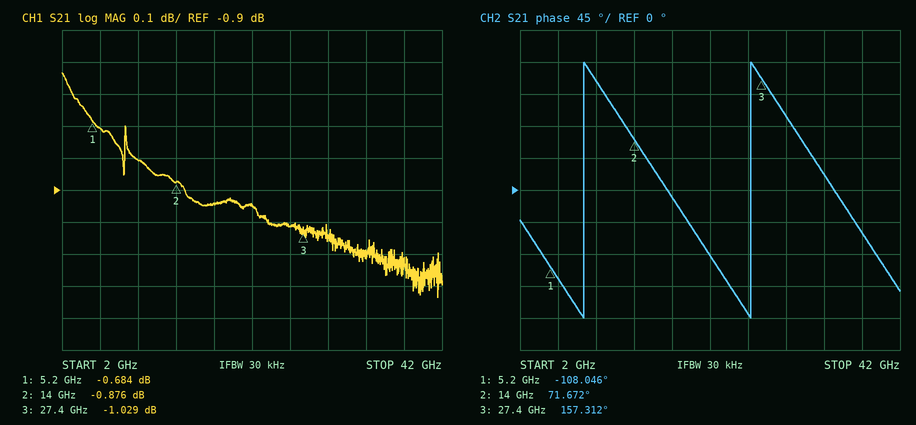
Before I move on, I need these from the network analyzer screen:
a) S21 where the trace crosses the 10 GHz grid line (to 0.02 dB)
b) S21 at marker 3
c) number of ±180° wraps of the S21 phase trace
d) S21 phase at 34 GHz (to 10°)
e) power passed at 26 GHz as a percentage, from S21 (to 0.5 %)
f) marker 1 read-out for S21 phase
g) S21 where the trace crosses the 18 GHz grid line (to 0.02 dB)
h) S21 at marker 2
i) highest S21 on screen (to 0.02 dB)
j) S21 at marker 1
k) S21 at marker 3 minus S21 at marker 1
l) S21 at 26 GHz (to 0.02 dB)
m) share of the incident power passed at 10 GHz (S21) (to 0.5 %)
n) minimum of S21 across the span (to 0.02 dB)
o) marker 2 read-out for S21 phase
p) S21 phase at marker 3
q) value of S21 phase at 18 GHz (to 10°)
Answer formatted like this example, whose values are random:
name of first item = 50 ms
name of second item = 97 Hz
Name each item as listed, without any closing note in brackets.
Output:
S21 where the trace crosses the 10 GHz grid line = -0.80 dB
S21 at marker 3 = -1.029 dB
number of ±180° wraps of the S21 phase trace = 2
S21 phase at 34 GHz = 20°
power passed at 26 GHz as a percentage, from S21 = 79.0 %
marker 1 read-out for S21 phase = -108.046°
S21 where the trace crosses the 18 GHz grid line = -0.94 dB
S21 at marker 2 = -0.876 dB
highest S21 on screen = -0.54 dB
S21 at marker 1 = -0.684 dB
S21 at marker 3 minus S21 at marker 1 = -0.345 dB
S21 at 26 GHz = -1.02 dB
share of the incident power passed at 10 GHz (S21) = 83.0 %
minimum of S21 across the span = -1.24 dB
marker 2 read-out for S21 phase = 71.672°
S21 phase at marker 3 = 157.312°
value of S21 phase at 18 GHz = -10°
